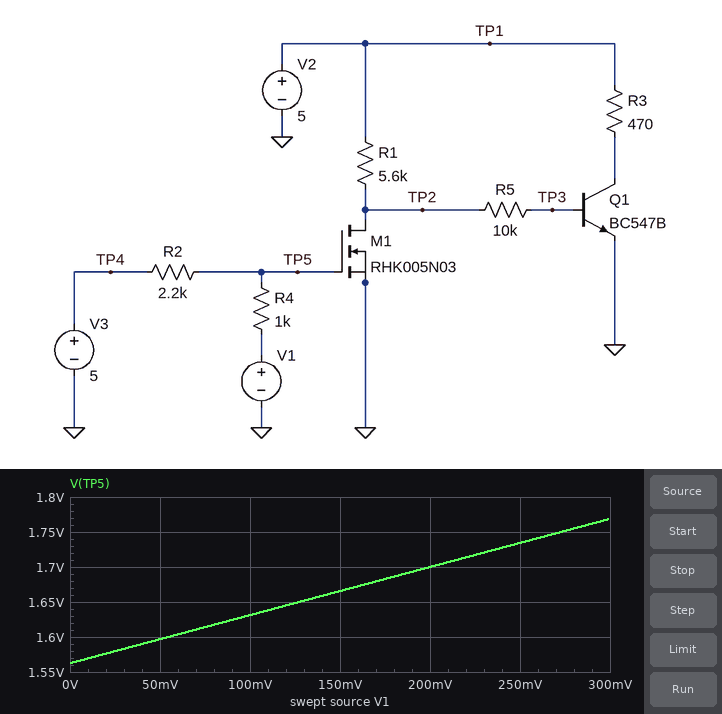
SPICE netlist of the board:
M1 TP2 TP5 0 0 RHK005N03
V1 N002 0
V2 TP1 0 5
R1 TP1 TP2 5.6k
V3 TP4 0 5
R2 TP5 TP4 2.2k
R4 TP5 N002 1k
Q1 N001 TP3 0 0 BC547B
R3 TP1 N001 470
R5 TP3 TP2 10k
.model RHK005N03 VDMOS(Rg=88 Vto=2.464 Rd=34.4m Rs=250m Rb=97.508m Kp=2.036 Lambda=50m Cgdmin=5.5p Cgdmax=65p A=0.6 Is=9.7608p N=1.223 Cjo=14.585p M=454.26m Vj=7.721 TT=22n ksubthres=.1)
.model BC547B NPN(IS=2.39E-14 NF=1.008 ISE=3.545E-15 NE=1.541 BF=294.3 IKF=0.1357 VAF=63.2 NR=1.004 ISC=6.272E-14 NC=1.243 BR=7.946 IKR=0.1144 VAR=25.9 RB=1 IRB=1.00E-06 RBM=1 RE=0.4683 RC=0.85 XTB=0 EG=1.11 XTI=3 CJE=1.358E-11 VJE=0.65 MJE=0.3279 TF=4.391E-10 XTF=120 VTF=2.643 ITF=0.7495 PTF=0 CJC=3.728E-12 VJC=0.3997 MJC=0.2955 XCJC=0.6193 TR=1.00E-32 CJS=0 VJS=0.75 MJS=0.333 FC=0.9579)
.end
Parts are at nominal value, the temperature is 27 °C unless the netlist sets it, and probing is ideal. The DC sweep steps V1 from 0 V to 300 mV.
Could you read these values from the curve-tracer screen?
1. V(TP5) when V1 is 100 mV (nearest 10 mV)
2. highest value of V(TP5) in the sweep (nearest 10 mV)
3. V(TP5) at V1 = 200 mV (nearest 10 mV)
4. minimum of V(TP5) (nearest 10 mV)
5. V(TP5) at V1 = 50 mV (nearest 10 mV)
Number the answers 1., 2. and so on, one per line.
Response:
1. 1.63 V
2. 1.77 V
3. 1.70 V
4. 1.56 V
5. 1.60 V
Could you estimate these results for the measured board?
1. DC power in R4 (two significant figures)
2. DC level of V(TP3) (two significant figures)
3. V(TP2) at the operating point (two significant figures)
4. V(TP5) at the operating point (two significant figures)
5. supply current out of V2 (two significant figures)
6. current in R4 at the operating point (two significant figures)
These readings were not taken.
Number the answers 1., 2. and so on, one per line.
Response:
1. 2.4 mW
2. 710 mV
3. 3.5 V
4. 1.6 V
5. 11 mA
6. 1.6 mA
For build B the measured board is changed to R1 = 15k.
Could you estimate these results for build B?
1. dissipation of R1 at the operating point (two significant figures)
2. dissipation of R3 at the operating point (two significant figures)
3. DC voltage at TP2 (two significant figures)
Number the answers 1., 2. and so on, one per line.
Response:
1. 440 µW
2. 51 mW
3. 2.4 V
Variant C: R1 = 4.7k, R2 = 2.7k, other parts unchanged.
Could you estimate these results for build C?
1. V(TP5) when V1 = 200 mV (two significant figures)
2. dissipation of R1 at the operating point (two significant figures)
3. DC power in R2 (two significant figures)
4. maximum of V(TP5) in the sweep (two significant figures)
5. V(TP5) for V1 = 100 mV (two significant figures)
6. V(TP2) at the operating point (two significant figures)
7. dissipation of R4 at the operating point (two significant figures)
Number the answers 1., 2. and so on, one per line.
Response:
1. 1.5 V
2. 400 µW
3. 4.9 mW
4. 1.6 V
5. 1.4 V
6. 3.6 V
7. 1.8 mW
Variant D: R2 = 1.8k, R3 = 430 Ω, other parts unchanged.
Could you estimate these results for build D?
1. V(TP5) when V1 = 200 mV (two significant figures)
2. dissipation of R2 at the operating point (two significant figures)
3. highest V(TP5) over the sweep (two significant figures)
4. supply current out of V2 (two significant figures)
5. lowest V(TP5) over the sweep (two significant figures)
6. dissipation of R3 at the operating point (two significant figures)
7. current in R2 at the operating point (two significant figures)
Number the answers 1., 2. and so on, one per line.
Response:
1. 1.9 V
2. 5.7 mW
3. 2.0 V
4. 12 mA
5. 1.8 V
6. 56 mW
7. 1.8 mA
